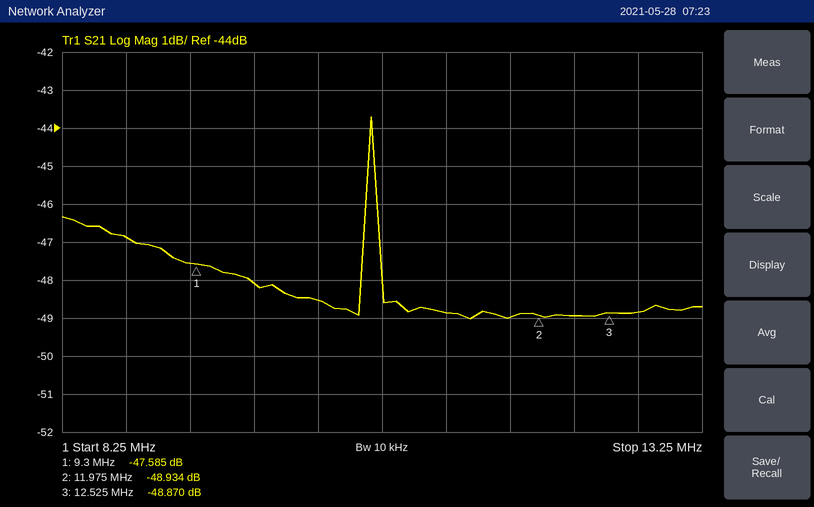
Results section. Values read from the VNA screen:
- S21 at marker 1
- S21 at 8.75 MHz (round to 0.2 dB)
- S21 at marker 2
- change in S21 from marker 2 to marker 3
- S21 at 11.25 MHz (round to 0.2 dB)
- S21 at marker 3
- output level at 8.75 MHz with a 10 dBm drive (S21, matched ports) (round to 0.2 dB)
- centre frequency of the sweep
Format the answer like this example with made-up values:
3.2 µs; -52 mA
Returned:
-47.585 dB; -46.8 dB; -48.934 dB; 0.064 dB; -48.8 dB; -48.870 dB; -36.8 dBm; 10.75 MHz
